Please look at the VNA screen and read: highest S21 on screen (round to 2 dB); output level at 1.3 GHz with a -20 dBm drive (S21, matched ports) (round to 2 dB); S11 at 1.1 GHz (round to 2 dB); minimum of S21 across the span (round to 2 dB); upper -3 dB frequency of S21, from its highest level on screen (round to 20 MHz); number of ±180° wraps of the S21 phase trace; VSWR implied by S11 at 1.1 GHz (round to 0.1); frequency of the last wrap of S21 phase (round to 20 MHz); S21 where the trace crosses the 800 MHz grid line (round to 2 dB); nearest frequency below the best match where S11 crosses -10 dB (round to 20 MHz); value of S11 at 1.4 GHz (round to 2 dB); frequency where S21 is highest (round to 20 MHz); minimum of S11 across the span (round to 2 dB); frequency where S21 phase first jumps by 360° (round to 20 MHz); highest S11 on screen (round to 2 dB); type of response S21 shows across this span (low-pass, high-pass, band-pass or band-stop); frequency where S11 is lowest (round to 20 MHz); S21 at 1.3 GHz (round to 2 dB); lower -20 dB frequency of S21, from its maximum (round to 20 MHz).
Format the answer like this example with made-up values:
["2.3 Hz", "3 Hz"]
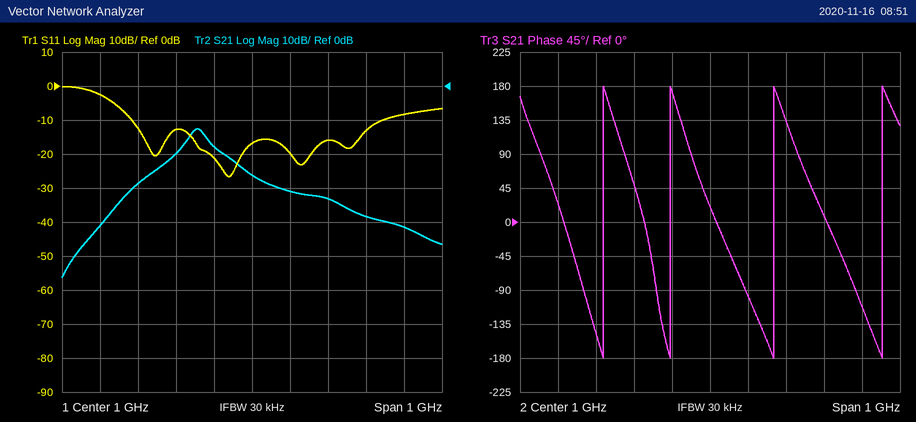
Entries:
["-12 dB", "-58 dBm", "-20 dB", "-56 dB", "880 MHz", "4", "1.2", "1.46 GHz", "-20 dB", "680 MHz", "-8 dB", "860 MHz", "-26 dB", "720 MHz", "0 dB", "band-pass", "940 MHz", "-38 dB", "660 MHz"]
